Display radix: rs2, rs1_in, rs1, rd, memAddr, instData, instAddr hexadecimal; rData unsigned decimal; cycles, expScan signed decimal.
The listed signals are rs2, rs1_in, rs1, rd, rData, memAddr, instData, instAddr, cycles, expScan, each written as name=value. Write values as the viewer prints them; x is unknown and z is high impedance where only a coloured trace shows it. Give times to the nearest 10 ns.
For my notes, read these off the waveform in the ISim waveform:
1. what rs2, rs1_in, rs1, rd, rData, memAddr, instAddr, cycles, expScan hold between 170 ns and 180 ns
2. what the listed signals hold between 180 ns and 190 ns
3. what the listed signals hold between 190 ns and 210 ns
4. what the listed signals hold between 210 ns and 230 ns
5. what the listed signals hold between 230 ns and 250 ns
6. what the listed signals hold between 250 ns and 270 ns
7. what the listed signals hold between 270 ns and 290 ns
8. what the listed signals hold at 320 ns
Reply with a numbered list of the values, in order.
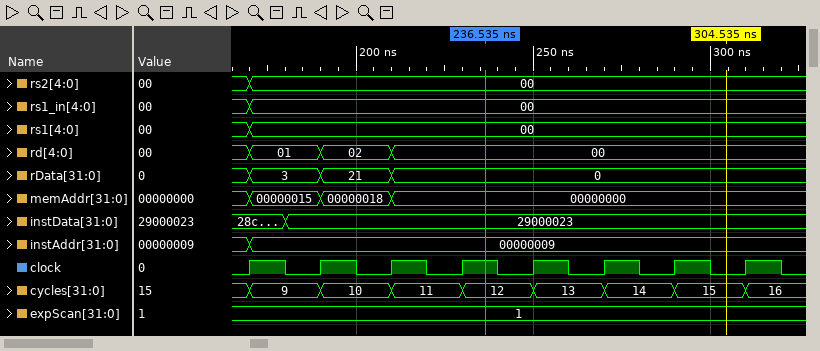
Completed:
1. rs2=00, rs1_in=00, rs1=00, rd=01, rData=3, memAddr=00000015, instAddr=00000009, cycles=9, expScan=1
2. rs2=00, rs1_in=00, rs1=00, rd=01, rData=3, memAddr=00000015, instData=29000023, instAddr=00000009, cycles=9, expScan=1
3. rs2=00, rs1_in=00, rs1=00, rd=02, rData=21, memAddr=00000018, instData=29000023, instAddr=00000009, cycles=10, expScan=1
4. rs2=00, rs1_in=00, rs1=00, rd=00, rData=0, memAddr=00000000, instData=29000023, instAddr=00000009, cycles=11, expScan=1
5. rs2=00, rs1_in=00, rs1=00, rd=00, rData=0, memAddr=00000000, instData=29000023, instAddr=00000009, cycles=12, expScan=1
6. rs2=00, rs1_in=00, rs1=00, rd=00, rData=0, memAddr=00000000, instData=29000023, instAddr=00000009, cycles=13, expScan=1
7. rs2=00, rs1_in=00, rs1=00, rd=00, rData=0, memAddr=00000000, instData=29000023, instAddr=00000009, cycles=14, expScan=1
8. rs2=00, rs1_in=00, rs1=00, rd=00, rData=0, memAddr=00000000, instData=29000023, instAddr=00000009, cycles=16, expScan=1
